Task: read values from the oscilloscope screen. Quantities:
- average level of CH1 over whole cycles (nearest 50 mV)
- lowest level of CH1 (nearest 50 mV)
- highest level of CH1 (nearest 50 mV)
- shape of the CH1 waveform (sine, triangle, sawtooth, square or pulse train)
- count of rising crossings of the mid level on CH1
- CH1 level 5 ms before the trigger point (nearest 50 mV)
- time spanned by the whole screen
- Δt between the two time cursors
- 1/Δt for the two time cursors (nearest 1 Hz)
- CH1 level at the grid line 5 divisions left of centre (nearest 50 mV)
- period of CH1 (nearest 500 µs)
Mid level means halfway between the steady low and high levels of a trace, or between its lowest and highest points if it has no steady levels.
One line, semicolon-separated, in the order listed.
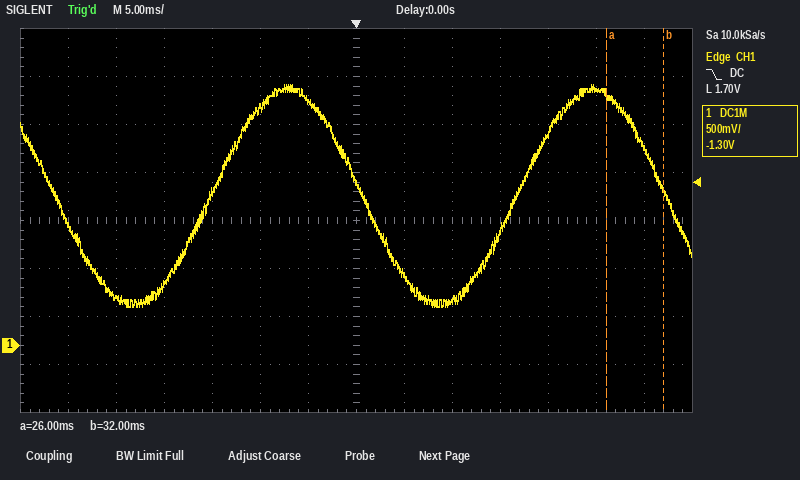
1.55 V; 400 mV; 2.70 V; sine; 2; 2.55 V; 70 ms; 6.0 ms; 167 Hz; 500 mV; 32.0 ms
